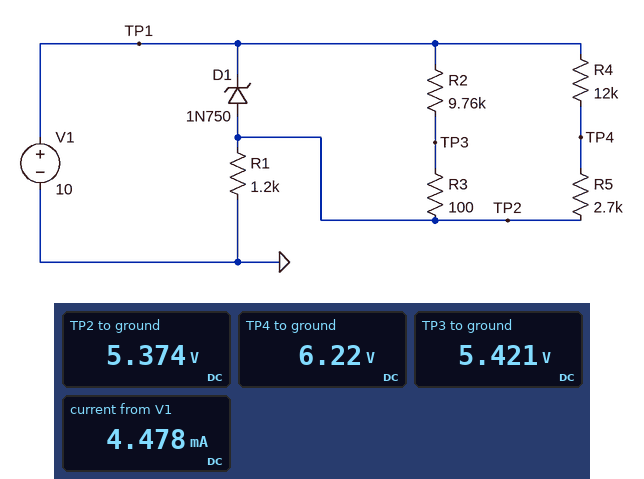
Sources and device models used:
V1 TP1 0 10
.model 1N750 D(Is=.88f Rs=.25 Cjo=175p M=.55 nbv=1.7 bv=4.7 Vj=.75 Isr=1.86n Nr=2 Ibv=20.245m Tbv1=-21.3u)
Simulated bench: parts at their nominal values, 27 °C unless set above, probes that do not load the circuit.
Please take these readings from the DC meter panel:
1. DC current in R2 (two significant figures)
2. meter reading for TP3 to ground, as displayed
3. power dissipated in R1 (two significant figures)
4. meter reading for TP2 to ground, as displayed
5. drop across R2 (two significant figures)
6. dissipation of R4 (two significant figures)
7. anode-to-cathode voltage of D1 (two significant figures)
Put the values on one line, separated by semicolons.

470 µA; 5.421 V; 24 mW; 5.374 V; 4.6 V; 1.2 mW; -4.6 V
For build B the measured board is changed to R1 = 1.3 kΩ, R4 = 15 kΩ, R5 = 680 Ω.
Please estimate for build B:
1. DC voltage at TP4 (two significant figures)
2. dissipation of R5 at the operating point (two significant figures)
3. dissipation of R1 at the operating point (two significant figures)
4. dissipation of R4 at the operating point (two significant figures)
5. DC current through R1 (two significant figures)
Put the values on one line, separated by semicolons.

5.6 V; 59 µW; 22 mW; 1.3 mW; 4.1 mA
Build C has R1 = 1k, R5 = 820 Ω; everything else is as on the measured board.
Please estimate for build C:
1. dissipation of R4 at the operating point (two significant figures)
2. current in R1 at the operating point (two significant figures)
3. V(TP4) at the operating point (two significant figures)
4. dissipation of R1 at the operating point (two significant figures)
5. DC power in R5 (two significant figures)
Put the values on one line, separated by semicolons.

1.6 mW; 5.4 mA; 5.7 V; 29 mW; 110 µW
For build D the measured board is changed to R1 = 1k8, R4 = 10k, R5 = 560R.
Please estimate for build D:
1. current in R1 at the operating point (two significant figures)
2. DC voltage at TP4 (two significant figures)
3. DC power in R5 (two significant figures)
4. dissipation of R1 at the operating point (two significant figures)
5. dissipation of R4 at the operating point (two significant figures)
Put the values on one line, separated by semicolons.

3.0 mA; 5.6 V; 110 µW; 16 mW; 1.9 mW
